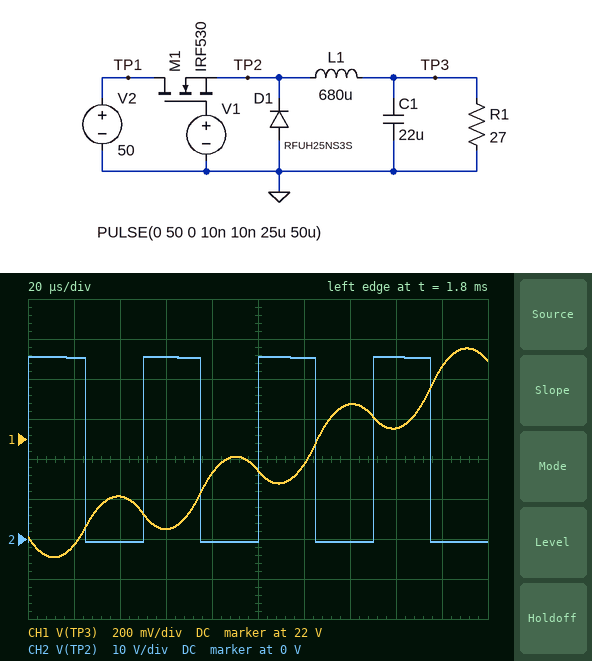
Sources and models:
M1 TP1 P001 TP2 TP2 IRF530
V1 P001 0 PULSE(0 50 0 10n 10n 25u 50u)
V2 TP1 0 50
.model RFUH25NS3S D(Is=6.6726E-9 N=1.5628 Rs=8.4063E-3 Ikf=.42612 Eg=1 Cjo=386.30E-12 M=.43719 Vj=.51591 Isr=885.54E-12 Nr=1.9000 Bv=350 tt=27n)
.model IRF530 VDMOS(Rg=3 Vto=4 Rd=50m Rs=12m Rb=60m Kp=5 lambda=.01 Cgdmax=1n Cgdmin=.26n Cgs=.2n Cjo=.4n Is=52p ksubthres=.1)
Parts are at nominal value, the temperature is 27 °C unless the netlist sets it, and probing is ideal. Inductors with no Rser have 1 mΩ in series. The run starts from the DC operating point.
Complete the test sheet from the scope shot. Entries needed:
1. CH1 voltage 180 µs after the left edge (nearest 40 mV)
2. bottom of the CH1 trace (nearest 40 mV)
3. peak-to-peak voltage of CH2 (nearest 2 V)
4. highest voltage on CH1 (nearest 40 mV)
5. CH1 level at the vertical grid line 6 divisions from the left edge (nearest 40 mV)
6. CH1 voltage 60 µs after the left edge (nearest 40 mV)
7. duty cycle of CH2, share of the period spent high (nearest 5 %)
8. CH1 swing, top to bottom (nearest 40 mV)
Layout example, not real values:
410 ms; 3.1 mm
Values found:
22.36 V; 21.40 V; 46 V; 22.44 V; 21.88 V; 21.56 V; 50 %; 1.04 V
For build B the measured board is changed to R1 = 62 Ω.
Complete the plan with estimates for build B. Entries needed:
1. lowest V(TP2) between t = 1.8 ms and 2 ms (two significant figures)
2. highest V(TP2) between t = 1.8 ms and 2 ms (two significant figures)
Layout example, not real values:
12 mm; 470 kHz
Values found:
-810 mV; 51 V
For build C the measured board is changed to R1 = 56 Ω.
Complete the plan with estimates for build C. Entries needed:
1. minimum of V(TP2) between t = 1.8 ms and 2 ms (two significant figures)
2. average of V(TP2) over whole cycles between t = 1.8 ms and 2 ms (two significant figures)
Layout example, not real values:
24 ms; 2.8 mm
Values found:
-810 mV; 24 V
